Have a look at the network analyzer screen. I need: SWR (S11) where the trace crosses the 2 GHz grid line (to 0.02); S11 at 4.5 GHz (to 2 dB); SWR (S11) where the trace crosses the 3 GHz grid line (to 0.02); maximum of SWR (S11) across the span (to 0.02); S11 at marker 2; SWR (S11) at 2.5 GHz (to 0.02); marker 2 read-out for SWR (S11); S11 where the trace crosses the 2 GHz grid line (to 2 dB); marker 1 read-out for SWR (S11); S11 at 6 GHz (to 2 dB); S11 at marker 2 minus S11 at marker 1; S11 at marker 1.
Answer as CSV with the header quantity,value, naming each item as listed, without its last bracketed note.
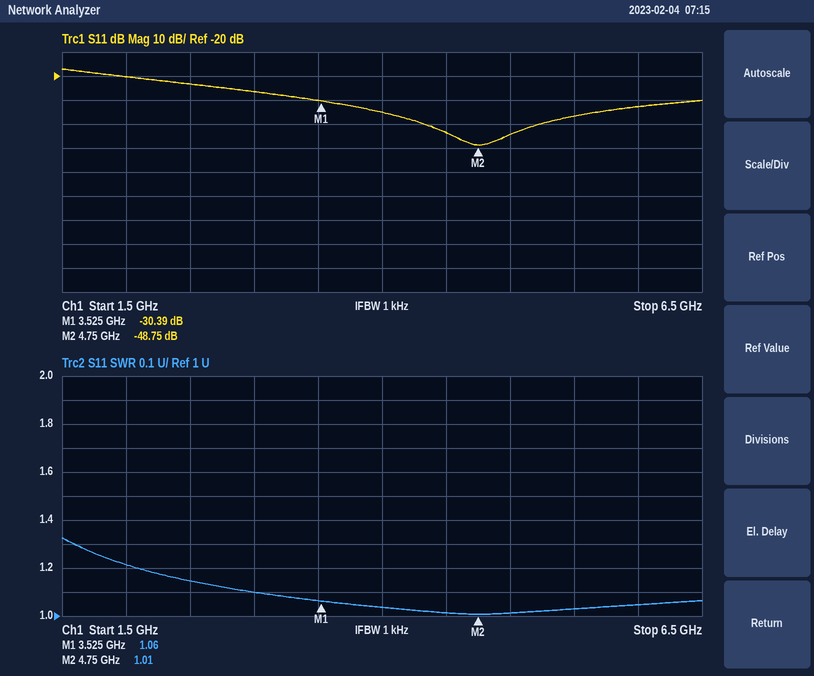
quantity,value
SWR (S11) where the trace crosses the 2 GHz grid line,1.22
S11 at 4.5 GHz,-44 dB
SWR (S11) where the trace crosses the 3 GHz grid line,1.10
maximum of SWR (S11) across the span,1.32
S11 at marker 2,-48.75 dB
SWR (S11) at 2.5 GHz,1.14
marker 2 read-out for SWR,1.01
S11 where the trace crosses the 2 GHz grid line,-20 dB
marker 1 read-out for SWR,1.06
S11 at 6 GHz,-32 dB
S11 at marker 2 minus S11 at marker 1,-18.36 dB
S11 at marker 1,-30.39 dB
